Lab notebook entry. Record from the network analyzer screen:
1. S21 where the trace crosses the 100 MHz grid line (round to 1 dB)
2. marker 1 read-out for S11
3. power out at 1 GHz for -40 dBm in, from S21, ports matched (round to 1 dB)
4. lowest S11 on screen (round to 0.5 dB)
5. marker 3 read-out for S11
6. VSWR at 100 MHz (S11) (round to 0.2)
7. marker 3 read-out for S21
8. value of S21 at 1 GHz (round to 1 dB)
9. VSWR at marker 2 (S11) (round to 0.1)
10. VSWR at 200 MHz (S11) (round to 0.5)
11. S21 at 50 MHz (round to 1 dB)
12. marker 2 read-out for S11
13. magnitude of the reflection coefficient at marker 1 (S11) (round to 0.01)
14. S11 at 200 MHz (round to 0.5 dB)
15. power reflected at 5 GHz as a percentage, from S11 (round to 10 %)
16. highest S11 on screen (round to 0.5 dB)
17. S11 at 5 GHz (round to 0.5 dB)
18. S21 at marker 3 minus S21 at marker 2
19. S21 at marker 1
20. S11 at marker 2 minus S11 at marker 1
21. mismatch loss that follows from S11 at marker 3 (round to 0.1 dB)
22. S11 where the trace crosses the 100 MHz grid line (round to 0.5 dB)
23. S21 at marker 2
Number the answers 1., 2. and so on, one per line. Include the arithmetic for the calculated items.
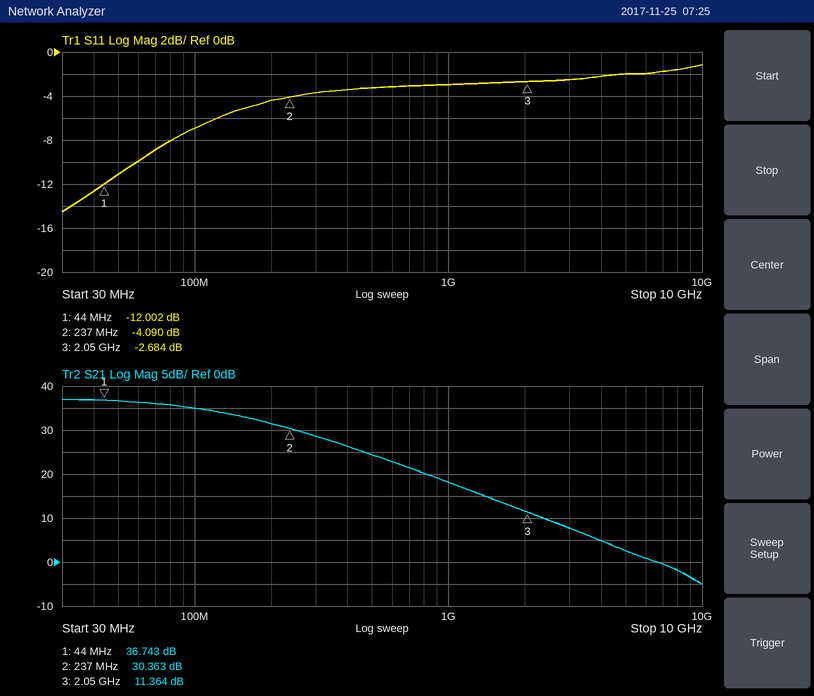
1. 35 dB
2. -12.002 dB
3. -40 dBm + (18 dB) = -22 dBm
4. -14.5 dB
5. -2.684 dB
6. |Γ| = 10^(-7/20) = 0.4467; VSWR = (1 + 0.4467)/(1 − 0.4467) ≈ 2.6
7. 11.364 dB
8. 18 dB
9. (1 + 0.6245)/(1 − 0.6245) ≈ 4.3
10. |Γ| = 10^(-4.5/20) = 0.5957; VSWR = (1 + 0.5957)/(1 − 0.5957) ≈ 4.0
11. 37 dB
12. -4.090 dB
13. 10^(-12.002/20) ≈ 0.25
14. -4.5 dB
15. 10^(-2/10) ≈ 63.1 %, so 60 % to the nearest 10 %
16. -1.0 dB
17. -2.0 dB
18. 11.364 − (30.363) = -18.999 dB
19. 36.743 dB
20. -4.09 − (-12.002) = 7.912 dB
21. −10 log10(1 − 10^(-2.684/10)) ≈ 3.4 dB
22. -7.0 dB
23. 30.363 dB
